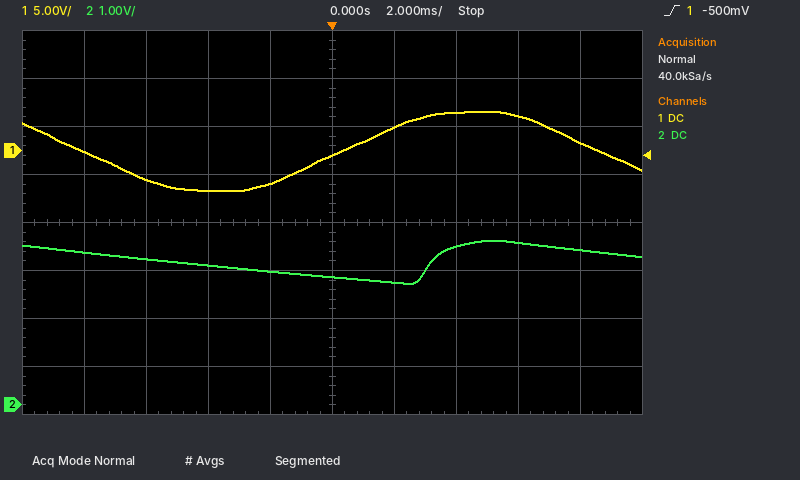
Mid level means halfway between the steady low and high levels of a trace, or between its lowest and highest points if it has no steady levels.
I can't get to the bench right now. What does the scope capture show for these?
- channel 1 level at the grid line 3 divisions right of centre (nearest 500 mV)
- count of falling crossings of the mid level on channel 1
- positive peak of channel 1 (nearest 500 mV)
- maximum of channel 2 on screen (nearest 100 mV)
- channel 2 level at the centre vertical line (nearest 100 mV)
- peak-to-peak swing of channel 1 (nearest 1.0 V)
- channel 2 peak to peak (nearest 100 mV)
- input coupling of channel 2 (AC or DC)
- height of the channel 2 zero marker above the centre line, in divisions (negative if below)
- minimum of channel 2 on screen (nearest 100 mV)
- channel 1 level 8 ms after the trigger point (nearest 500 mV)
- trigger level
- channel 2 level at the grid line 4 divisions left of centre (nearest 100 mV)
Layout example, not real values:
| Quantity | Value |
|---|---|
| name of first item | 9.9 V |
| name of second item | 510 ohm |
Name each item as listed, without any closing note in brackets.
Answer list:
| Quantity | Value |
|---|---|
| channel 1 level at the grid line 3 divisions right of centre | 3.5 V |
| count of falling crossings of the mid level on channel 1 | 2 |
| positive peak of channel 1 | 4.0 V |
| maximum of channel 2 on screen | 3.4 V |
| channel 2 level at the centre vertical line | 2.7 V |
| peak-to-peak swing of channel 1 | 8.0 V |
| channel 2 peak to peak | 900 mV |
| input coupling of channel 2 | DC |
| height of the channel 2 zero marker above the centre line, in divisions | -3.8 div |
| minimum of channel 2 on screen | 2.5 V |
| channel 1 level 8 ms after the trigger point | 1.0 V |
| trigger level | -500 mV |
| channel 2 level at the grid line 4 divisions left of centre | 3.2 V |
